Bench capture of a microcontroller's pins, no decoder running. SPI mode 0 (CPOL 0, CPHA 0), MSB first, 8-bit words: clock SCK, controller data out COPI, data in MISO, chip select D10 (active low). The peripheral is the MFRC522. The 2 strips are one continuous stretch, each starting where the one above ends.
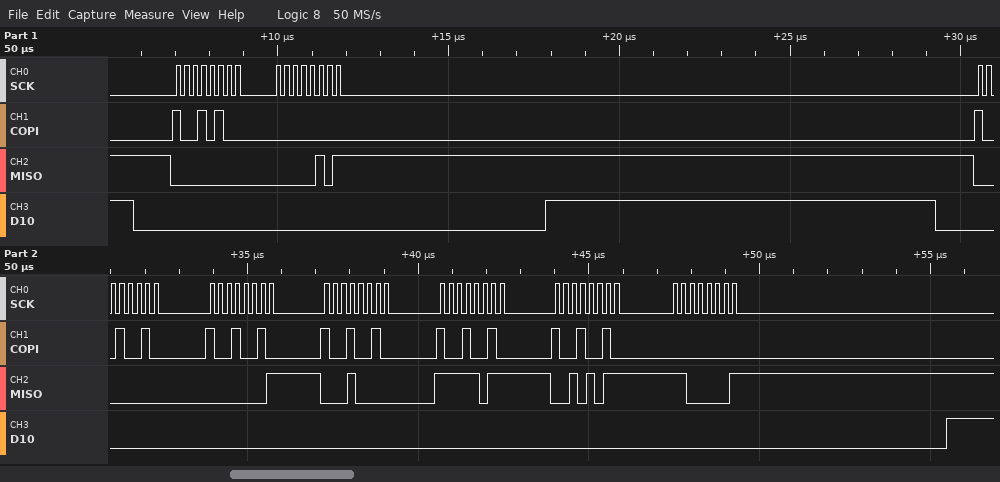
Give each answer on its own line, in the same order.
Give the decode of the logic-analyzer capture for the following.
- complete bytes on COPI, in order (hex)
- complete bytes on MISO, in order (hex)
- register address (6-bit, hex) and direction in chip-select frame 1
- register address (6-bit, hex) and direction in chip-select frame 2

94 00 92 92 92 92 92 00
00 05 00 01 10 FB 2B C1
0x0A read
0x09 read
